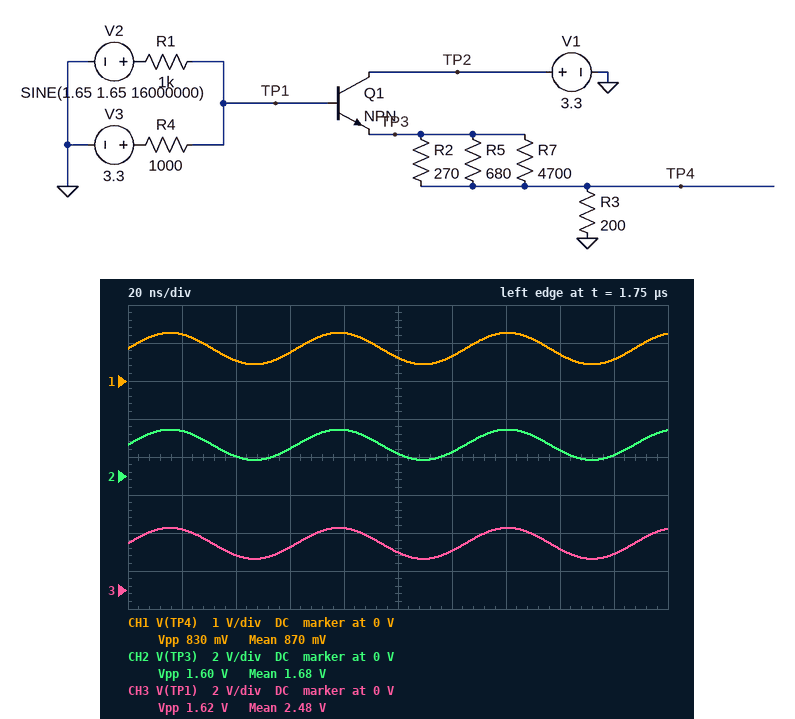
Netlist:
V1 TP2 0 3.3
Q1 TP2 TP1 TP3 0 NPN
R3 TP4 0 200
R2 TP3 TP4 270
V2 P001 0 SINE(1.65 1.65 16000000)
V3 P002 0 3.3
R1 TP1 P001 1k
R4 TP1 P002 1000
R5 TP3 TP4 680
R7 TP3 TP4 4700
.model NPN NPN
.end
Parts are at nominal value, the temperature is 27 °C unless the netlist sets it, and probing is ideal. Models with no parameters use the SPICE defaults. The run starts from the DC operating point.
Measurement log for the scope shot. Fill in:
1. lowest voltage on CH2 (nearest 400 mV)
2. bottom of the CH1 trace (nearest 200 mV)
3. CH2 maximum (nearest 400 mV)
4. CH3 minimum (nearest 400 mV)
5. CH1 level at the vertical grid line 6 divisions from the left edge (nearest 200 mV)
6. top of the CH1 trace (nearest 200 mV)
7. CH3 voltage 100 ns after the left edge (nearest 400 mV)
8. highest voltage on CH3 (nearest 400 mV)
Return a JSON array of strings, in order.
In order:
["800 mV", "400 mV", "2.4 V", "1.6 V", "600 mV", "1.2 V", "2.0 V", "3.2 V"]
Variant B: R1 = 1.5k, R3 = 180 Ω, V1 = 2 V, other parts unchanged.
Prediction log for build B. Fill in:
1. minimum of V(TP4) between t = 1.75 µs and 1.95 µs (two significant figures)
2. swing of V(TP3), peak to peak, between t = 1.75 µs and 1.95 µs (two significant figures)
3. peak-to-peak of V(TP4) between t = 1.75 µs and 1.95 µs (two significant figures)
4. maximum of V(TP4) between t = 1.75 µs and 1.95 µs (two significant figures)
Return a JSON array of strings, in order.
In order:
["570 mV", "790 mV", "390 mV", "960 mV"]
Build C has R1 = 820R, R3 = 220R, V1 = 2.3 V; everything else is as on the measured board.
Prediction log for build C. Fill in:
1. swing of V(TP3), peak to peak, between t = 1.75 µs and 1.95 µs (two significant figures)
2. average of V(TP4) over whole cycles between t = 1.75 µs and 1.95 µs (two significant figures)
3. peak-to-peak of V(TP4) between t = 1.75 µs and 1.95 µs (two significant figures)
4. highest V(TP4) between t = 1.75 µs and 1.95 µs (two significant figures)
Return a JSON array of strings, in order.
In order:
["1.5 V", "830 mV", "840 mV", "1.2 V"]
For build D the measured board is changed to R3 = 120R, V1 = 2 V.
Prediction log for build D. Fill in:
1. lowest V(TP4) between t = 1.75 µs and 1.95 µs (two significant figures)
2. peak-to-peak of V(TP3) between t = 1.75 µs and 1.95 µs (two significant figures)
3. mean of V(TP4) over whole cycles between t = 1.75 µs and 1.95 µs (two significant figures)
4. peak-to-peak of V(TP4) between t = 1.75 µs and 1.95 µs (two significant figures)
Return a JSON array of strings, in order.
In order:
["330 mV", "1.1 V", "590 mV", "440 mV"]
